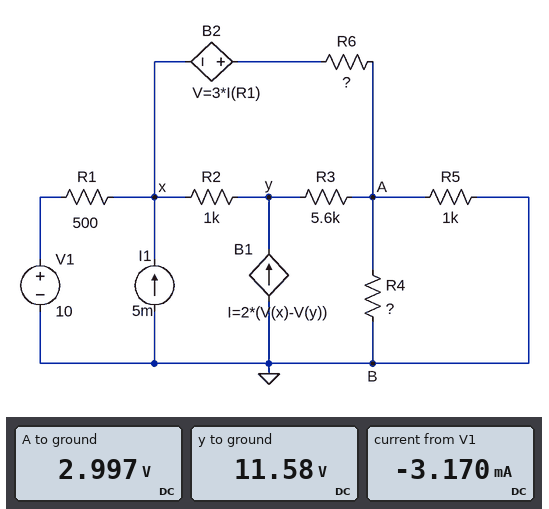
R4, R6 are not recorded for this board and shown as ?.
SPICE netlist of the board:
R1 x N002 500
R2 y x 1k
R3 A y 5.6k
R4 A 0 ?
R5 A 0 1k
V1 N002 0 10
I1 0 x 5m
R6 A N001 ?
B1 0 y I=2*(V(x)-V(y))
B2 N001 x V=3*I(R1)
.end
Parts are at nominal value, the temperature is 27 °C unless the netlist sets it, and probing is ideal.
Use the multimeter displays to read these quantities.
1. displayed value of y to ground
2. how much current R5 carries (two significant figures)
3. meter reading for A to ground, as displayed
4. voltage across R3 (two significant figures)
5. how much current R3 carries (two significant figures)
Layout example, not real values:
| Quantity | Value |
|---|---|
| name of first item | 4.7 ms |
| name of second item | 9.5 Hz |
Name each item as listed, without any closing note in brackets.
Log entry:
| Quantity | Value |
|---|---|
| displayed value of y to ground | 11.58 V |
| how much current R5 carries | 3.0 mA |
| meter reading for A to ground, as displayed | 2.997 V |
| voltage across R3 | 8.6 V |
| how much current R3 carries | 1.5 mA |
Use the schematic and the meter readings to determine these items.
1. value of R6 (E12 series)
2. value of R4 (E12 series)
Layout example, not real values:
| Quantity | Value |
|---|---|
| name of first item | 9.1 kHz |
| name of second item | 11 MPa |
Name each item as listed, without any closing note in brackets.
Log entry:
| Quantity | Value |
|---|---|
| value of R6 | 4.7 kΩ |
| value of R4 | 8.2 kΩ |
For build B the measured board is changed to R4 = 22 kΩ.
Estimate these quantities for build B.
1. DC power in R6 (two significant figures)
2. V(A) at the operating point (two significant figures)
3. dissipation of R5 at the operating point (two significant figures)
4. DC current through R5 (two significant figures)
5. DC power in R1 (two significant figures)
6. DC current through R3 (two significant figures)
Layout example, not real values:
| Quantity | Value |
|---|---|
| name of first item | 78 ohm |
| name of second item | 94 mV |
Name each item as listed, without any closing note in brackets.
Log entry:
| Quantity | Value |
|---|---|
| DC power in R6 | 15 mW |
| V(A) at the operating point | 3.2 V |
| dissipation of R5 at the operating point | 10 mW |
| DC current through R5 | 3.2 mA |
| DC power in R1 | 5.1 mW |
| DC current through R3 | 1.5 mA |
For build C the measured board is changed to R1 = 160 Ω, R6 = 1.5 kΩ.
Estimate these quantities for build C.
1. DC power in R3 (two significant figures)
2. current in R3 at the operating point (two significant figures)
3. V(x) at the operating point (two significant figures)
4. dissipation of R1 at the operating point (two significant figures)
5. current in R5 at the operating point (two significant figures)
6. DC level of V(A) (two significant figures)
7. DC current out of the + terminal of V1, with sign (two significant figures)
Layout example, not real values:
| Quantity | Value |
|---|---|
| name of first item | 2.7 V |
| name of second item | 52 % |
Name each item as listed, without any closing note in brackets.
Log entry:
| Quantity | Value |
|---|---|
| DC power in R3 | 6.0 mW |
| current in R3 at the operating point | 1.0 mA |
| V(x) at the operating point | 10 V |
| dissipation of R1 at the operating point | 200 µW |
| current in R5 at the operating point | 4.4 mA |
| DC level of V(A) | 4.4 V |
| DC current out of the + terminal of V1, with sign | -1.1 mA |
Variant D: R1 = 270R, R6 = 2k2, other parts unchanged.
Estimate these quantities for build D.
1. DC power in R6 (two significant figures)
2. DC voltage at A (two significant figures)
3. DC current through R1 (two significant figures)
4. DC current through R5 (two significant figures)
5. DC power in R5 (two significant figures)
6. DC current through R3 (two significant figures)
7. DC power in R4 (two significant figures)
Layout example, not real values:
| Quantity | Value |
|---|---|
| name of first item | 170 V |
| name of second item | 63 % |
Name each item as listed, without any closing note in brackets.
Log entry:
| Quantity | Value |
|---|---|
| DC power in R6 | 21 mW |
| DC voltage at A | 3.8 V |
| DC current through R1 | 1.9 mA |
| DC current through R5 | 3.8 mA |
| DC power in R5 | 14 mW |
| DC current through R3 | 1.2 mA |
| DC power in R4 | 1.8 mW |
